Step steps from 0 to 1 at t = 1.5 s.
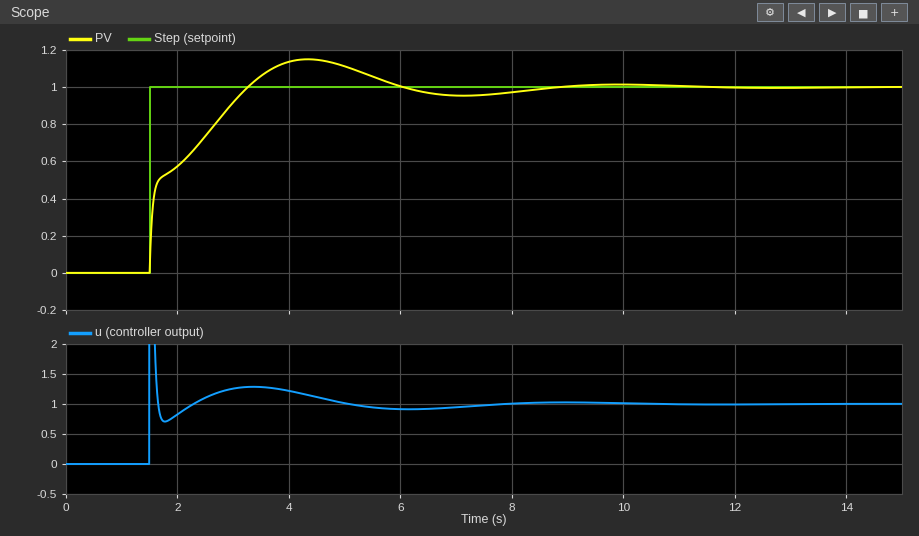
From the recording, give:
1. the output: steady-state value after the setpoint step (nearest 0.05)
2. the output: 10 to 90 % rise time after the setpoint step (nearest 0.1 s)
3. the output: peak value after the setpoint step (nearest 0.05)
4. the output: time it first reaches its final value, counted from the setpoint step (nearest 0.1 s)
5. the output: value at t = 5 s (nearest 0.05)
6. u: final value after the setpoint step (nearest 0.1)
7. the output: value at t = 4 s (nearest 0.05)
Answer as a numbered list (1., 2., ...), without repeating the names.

1. 1.00
2. 1.4 s
3. 1.15
4. 1.8 s
5. 1.10
6. 1.0
7. 1.15
